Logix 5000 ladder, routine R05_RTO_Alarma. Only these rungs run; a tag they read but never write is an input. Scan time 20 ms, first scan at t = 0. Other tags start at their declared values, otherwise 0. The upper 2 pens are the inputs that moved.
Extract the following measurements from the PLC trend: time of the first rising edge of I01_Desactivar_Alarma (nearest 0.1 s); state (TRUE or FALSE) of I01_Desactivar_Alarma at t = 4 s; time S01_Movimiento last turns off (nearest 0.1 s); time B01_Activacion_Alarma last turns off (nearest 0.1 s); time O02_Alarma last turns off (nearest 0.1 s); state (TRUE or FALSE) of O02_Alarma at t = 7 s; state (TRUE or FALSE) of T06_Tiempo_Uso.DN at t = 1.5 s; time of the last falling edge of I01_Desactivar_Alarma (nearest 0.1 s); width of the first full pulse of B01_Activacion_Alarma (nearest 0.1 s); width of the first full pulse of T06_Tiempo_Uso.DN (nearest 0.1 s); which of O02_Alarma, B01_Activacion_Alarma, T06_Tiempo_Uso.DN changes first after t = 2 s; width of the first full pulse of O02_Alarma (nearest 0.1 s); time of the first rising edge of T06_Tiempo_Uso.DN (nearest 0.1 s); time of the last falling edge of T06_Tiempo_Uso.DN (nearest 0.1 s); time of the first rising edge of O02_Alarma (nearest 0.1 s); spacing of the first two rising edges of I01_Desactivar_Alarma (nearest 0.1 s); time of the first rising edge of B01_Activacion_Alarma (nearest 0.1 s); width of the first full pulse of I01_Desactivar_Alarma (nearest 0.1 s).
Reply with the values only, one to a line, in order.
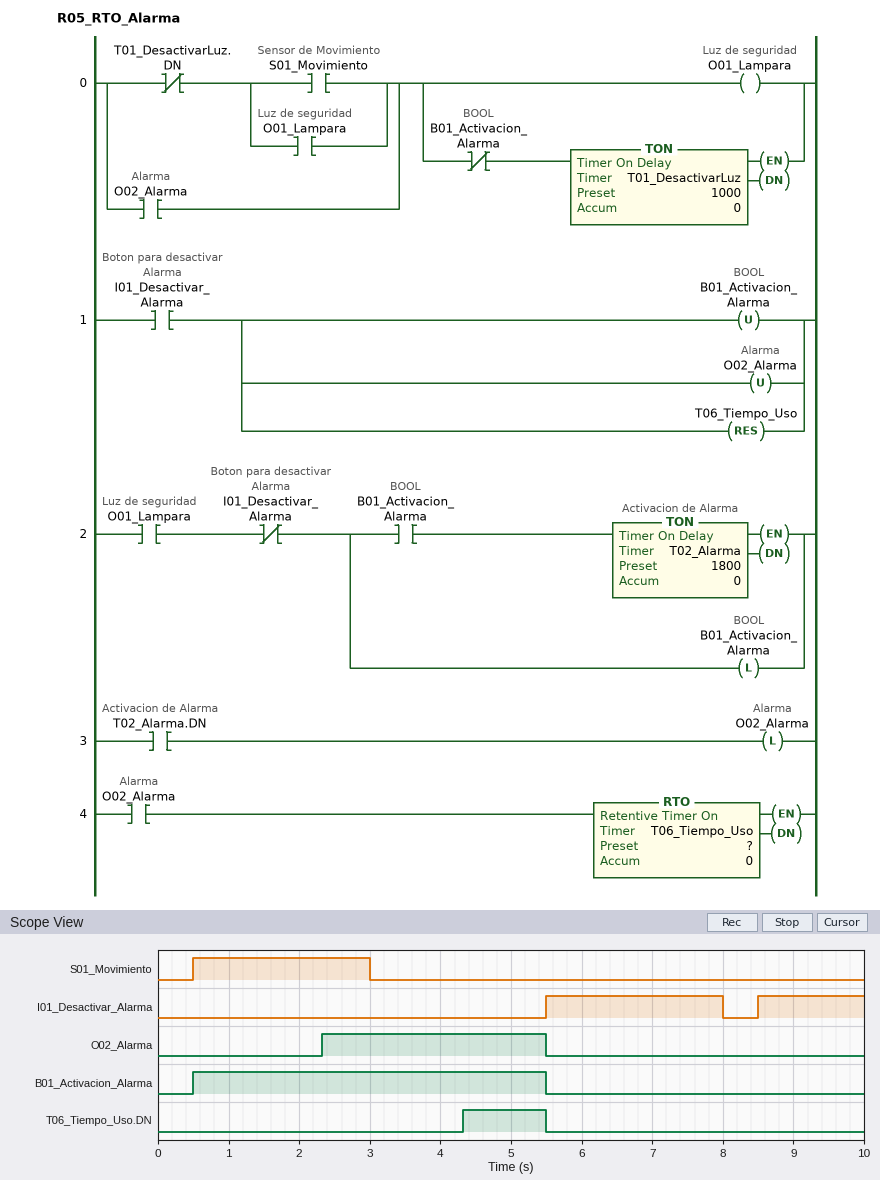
5.5 s
FALSE
3.0 s
5.5 s
5.5 s
FALSE
FALSE
8.0 s
5.0 s
1.2 s
O02_Alarma
3.2 s
4.3 s
5.5 s
2.3 s
3.0 s
0.5 s
2.5 s
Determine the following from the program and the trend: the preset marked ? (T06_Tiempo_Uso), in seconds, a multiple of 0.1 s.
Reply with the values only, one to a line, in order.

2.0 s
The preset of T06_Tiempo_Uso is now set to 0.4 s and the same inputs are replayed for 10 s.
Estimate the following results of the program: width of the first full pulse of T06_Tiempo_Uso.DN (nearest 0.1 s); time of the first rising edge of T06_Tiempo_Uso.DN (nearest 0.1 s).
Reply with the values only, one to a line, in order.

2.8 s
2.7 s
